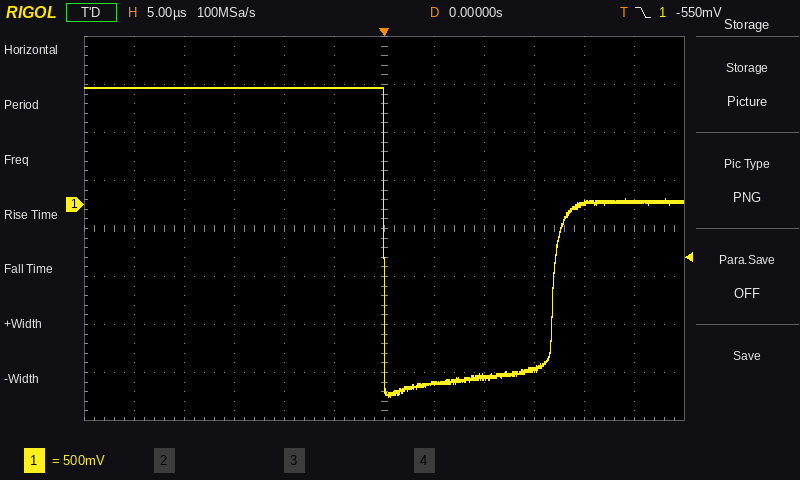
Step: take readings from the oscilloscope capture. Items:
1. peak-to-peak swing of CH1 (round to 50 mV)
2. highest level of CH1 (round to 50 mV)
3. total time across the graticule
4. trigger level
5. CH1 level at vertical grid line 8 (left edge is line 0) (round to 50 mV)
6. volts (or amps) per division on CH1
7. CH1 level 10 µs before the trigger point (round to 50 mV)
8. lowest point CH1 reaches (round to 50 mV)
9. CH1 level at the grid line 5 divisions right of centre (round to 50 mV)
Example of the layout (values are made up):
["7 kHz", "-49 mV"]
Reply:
["3.20 V", "1.20 V", "60 µs", "-550 mV", "-1.80 V", "500 mV", "1.20 V", "-2.00 V", "50 mV"]
